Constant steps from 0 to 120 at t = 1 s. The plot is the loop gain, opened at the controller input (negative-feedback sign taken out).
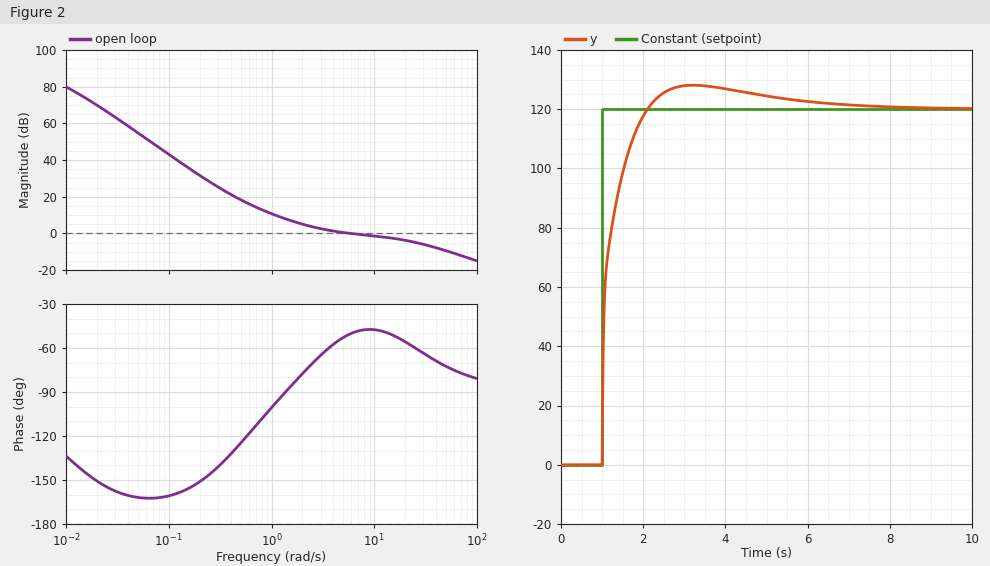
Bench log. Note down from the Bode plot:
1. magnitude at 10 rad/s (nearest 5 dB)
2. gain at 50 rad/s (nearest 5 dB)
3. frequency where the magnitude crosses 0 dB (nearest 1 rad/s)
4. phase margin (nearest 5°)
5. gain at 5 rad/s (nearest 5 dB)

0 dB
-10 dB
6 rad/s
130°
0 dB
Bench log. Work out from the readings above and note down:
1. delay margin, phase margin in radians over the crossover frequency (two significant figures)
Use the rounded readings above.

0.38 s
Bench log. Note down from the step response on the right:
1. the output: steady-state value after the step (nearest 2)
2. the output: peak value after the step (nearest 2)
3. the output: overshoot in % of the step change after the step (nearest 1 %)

120
128
7 %
